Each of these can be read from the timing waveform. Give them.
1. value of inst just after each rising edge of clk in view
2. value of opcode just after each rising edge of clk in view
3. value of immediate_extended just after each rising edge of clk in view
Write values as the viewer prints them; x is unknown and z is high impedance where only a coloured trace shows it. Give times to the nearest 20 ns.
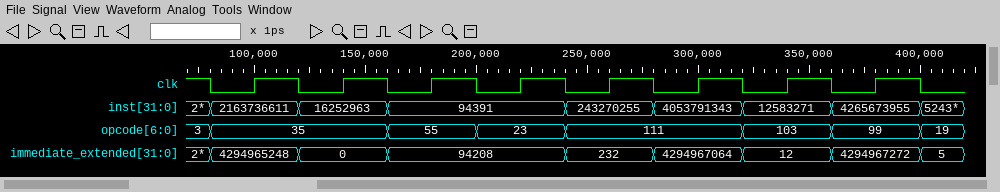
2163736611, 16252963, 94391, 94391, 243270255, 4053791343, 12583271, 4265673955
35, 35, 55, 23, 111, 111, 103, 99
4294965248, 0, 94208, 94208, 232, 4294967064, 12, 4294967272
